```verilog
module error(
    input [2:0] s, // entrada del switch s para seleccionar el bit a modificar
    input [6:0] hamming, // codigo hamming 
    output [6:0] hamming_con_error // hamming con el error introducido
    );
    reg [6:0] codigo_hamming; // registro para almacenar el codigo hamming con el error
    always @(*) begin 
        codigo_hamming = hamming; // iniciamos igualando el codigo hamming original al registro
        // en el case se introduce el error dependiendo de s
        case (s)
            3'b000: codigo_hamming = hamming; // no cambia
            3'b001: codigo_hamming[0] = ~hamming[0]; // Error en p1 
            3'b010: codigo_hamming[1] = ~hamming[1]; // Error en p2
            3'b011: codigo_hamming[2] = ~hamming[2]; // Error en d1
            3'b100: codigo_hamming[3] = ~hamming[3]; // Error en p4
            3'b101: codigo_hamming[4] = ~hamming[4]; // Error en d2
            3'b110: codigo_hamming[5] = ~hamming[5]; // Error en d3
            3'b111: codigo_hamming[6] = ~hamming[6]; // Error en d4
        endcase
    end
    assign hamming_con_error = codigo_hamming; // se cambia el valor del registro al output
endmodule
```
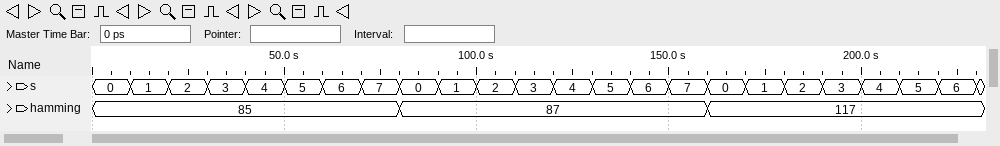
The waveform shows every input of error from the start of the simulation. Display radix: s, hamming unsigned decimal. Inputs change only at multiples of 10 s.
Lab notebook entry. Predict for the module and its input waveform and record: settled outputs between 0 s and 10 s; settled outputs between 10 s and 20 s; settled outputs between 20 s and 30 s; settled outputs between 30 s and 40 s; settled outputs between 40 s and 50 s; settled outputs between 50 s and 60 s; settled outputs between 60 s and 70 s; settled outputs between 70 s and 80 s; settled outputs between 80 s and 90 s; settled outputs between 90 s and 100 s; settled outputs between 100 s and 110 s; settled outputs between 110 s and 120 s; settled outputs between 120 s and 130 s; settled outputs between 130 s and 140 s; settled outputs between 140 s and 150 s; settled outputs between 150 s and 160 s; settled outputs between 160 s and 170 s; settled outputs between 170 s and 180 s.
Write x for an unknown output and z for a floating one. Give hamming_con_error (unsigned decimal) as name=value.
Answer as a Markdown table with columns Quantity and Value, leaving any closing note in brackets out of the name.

| Quantity | Value |
|---|---|
| settled outputs between 0 s and 10 s | hamming_con_error=85 |
| settled outputs between 10 s and 20 s | hamming_con_error=84 |
| settled outputs between 20 s and 30 s | hamming_con_error=87 |
| settled outputs between 30 s and 40 s | hamming_con_error=81 |
| settled outputs between 40 s and 50 s | hamming_con_error=93 |
| settled outputs between 50 s and 60 s | hamming_con_error=69 |
| settled outputs between 60 s and 70 s | hamming_con_error=117 |
| settled outputs between 70 s and 80 s | hamming_con_error=21 |
| settled outputs between 80 s and 90 s | hamming_con_error=87 |
| settled outputs between 90 s and 100 s | hamming_con_error=86 |
| settled outputs between 100 s and 110 s | hamming_con_error=85 |
| settled outputs between 110 s and 120 s | hamming_con_error=83 |
| settled outputs between 120 s and 130 s | hamming_con_error=95 |
| settled outputs between 130 s and 140 s | hamming_con_error=71 |
| settled outputs between 140 s and 150 s | hamming_con_error=119 |
| settled outputs between 150 s and 160 s | hamming_con_error=23 |
| settled outputs between 160 s and 170 s | hamming_con_error=117 |
| settled outputs between 170 s and 180 s | hamming_con_error=116 |
